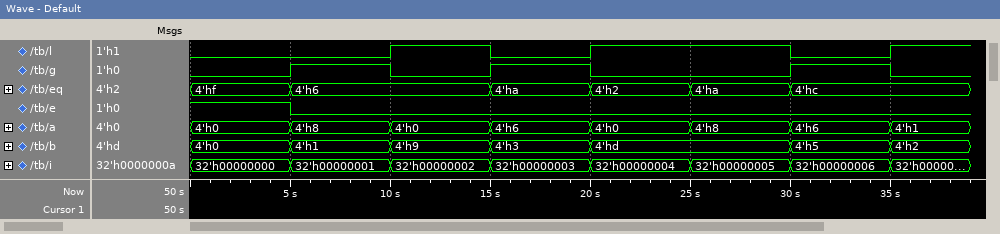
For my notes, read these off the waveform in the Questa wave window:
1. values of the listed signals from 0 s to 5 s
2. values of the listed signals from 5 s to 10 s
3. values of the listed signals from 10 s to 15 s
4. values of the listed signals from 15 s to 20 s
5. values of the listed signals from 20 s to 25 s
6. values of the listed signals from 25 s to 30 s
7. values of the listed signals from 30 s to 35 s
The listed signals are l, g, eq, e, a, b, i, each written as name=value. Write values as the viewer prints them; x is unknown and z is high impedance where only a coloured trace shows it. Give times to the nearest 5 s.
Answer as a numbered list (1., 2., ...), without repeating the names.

1. l=0, g=0, eq=4'hf, e=1, a=4'h0, b=4'h0, i=32'h00000000
2. l=0, g=1, eq=4'h6, e=0, a=4'h8, b=4'h1, i=32'h00000001
3. l=1, g=0, eq=4'h6, e=0, a=4'h0, b=4'h9, i=32'h00000002
4. l=0, g=1, eq=4'ha, e=0, a=4'h6, b=4'h3, i=32'h00000003
5. l=1, g=0, eq=4'h2, e=0, a=4'h0, b=4'hd, i=32'h00000004
6. l=1, g=0, eq=4'ha, e=0, a=4'h8, b=4'hd, i=32'h00000005
7. l=0, g=1, eq=4'hc, e=0, a=4'h6, b=4'h5, i=32'h00000006
